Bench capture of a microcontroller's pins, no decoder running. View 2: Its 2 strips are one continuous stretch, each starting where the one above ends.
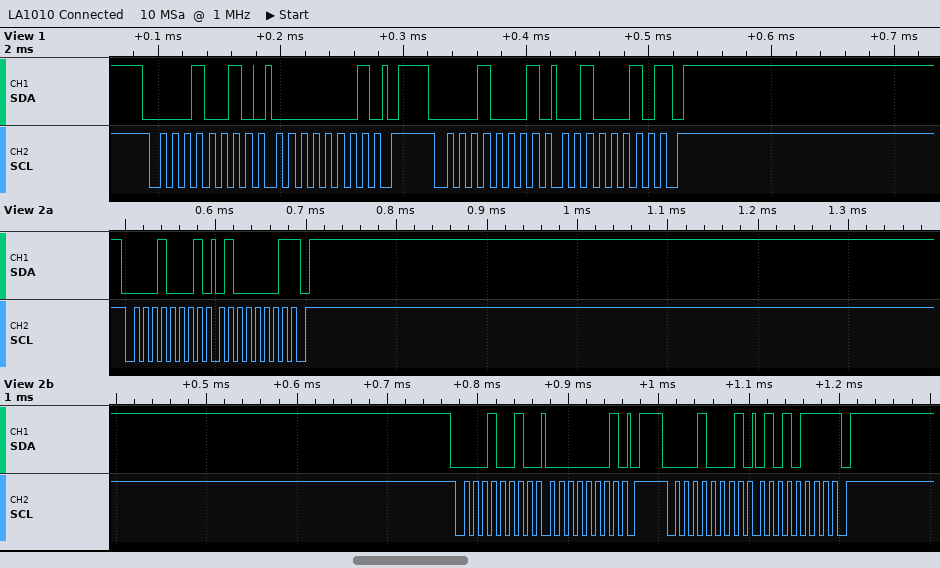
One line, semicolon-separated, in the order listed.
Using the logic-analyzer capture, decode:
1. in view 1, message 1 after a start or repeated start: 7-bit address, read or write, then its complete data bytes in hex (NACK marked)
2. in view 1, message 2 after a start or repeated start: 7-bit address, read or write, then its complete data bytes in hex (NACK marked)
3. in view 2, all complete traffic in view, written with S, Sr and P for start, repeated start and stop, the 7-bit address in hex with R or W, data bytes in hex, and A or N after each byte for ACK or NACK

0x09 write: 01; 0x08 read: 22 NACK; S 08R A 41 N P S 09W A 01 A P S 08R A 57 N P
